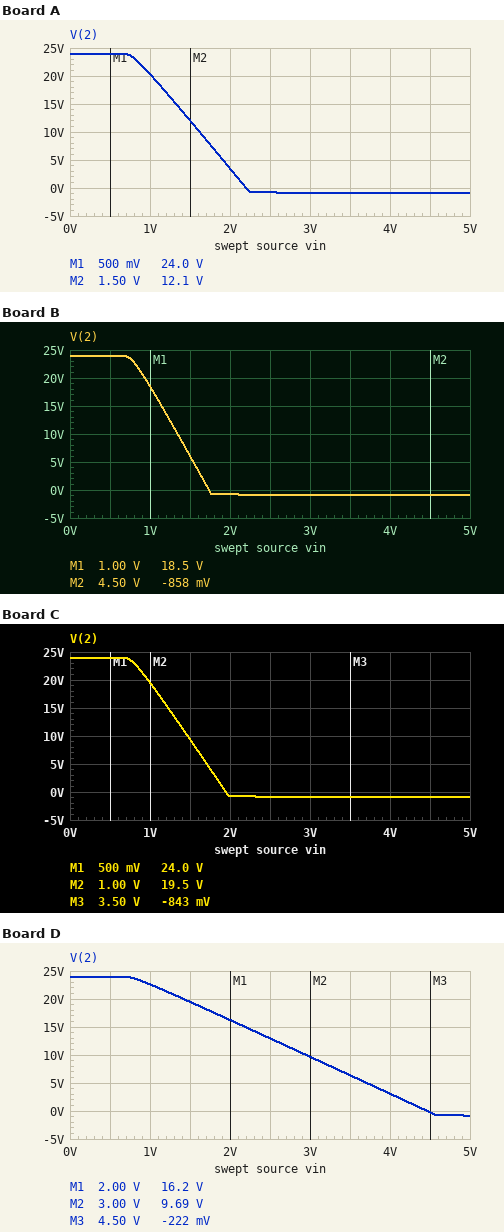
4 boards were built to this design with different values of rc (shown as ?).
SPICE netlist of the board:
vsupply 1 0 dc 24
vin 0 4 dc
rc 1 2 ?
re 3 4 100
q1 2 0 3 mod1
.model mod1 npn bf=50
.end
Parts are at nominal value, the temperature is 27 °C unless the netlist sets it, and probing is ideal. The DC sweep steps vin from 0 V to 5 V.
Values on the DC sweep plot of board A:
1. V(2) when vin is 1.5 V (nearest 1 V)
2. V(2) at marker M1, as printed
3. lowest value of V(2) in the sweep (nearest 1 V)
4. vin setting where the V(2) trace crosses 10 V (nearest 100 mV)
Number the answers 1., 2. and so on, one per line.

1. 12 V
2. 24.0 V
3. -1 V
4. 1.6 V
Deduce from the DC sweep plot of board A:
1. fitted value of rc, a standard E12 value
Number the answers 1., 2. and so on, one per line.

1. 1.8 kΩ
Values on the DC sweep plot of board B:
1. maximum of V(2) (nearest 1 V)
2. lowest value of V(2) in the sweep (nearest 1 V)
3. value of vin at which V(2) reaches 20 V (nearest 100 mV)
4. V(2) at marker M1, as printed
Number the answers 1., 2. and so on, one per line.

1. 24 V
2. -1 V
3. 900 mV
4. 18.5 V
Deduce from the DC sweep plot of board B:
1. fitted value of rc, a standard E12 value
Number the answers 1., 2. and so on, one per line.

1. 2.7 kΩ
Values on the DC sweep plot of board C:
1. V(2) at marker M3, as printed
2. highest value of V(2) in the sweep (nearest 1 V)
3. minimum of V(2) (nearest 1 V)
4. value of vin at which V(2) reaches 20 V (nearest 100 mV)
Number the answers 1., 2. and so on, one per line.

1. -843 mV
2. 24 V
3. -1 V
4. 1.0 V
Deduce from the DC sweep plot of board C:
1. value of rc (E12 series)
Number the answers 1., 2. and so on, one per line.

1. 2.2 kΩ
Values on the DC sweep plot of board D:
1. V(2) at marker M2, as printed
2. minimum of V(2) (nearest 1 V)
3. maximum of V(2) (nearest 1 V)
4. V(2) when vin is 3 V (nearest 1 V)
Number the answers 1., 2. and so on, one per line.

1. 9.69 V
2. -1 V
3. 24 V
4. 10 V
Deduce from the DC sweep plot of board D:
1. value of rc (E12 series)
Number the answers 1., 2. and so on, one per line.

1. 680 Ω
